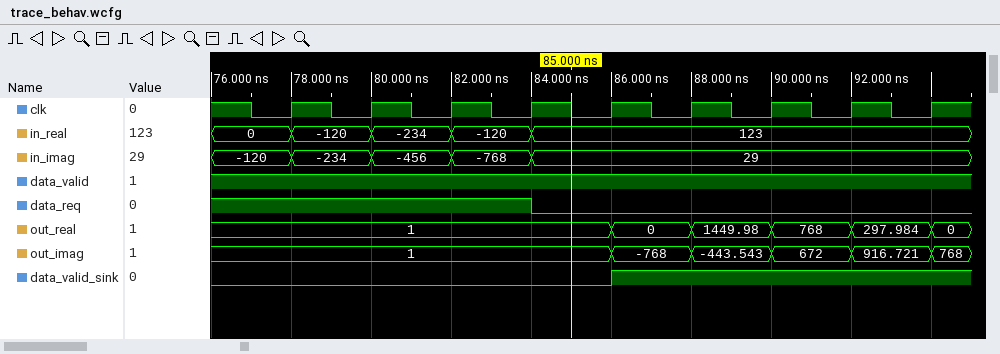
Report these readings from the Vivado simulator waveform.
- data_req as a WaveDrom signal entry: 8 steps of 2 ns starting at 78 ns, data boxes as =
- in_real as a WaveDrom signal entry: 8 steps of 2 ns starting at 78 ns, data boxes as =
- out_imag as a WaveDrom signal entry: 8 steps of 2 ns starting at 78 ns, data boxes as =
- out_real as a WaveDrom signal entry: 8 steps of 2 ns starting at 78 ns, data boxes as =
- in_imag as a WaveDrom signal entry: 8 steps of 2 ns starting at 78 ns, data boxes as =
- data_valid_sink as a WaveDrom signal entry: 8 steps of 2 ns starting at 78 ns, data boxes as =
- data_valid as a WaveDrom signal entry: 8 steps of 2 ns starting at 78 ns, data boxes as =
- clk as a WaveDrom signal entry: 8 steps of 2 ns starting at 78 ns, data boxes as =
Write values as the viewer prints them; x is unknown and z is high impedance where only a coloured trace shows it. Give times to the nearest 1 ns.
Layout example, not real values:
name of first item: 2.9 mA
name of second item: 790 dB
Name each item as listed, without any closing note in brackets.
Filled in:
data_req as a WaveDrom signal entry: 8 steps of 2 ns starting at 78 ns, data boxes as =: {name: 'data_req', wave: '1..0....'}
in_real as a WaveDrom signal entry: 8 steps of 2 ns starting at 78 ns, data boxes as =: {name: 'in_real', wave: '====....', data: '-120 -234 -120 123'}
out_imag as a WaveDrom signal entry: 8 steps of 2 ns starting at 78 ns, data boxes as =: {name: 'out_imag', wave: '=...====', data: '1 -768 -443.543 672 916.721'}
out_real as a WaveDrom signal entry: 8 steps of 2 ns starting at 78 ns, data boxes as =: {name: 'out_real', wave: '=...====', data: '1 0 1449.98 768 297.984'}
in_imag as a WaveDrom signal entry: 8 steps of 2 ns starting at 78 ns, data boxes as =: {name: 'in_imag', wave: '====....', data: '-234 -456 -768 29'}
data_valid_sink as a WaveDrom signal entry: 8 steps of 2 ns starting at 78 ns, data boxes as =: {name: 'data_valid_sink', wave: '0...1...'}
data_valid as a WaveDrom signal entry: 8 steps of 2 ns starting at 78 ns, data boxes as =: {name: 'data_valid', wave: '1.......'}
clk as a WaveDrom signal entry: 8 steps of 2 ns starting at 78 ns, data boxes as =: {name: 'clk', wave: 'p.......'}
